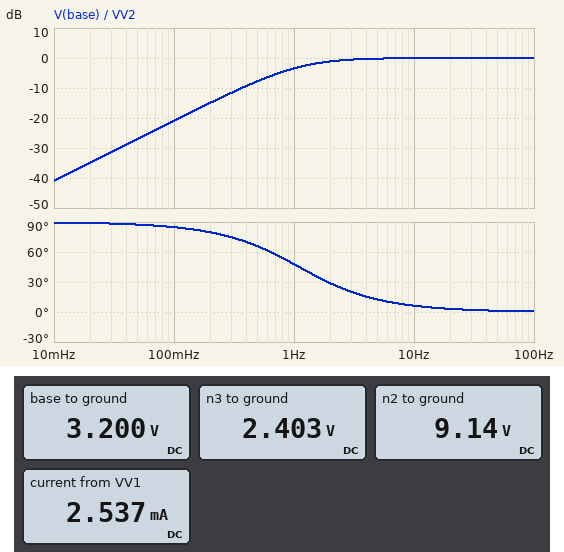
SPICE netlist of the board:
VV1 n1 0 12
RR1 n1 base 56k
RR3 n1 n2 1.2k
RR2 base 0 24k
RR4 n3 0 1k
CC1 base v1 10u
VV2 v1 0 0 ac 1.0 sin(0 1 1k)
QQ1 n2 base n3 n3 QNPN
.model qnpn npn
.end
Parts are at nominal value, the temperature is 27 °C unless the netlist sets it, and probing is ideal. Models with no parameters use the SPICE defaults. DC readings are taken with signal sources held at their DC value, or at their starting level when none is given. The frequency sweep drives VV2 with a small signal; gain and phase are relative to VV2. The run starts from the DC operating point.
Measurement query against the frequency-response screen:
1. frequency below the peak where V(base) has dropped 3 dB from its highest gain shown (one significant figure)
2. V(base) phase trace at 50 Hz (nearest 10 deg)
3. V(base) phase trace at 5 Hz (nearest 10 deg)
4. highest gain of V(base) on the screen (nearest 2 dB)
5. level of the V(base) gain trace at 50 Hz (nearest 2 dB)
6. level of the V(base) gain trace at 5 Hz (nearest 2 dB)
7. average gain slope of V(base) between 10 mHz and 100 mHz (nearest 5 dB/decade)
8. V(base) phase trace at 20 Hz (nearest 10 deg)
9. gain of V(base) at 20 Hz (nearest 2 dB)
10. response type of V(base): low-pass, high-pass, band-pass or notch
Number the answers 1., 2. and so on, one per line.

1. 1 Hz
2. 0 deg
3. 10 deg
4. 0 dB
5. 0 dB
6. 0 dB
7. 20 dB/decade
8. 0 deg
9. 0 dB
10. high-pass
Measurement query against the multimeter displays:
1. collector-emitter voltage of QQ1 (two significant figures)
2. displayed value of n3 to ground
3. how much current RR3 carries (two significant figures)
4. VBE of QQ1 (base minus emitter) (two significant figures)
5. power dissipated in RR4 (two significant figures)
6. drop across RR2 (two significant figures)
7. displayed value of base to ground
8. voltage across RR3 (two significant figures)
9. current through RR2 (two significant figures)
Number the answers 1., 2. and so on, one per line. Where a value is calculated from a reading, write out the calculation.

1. 9.14 V - 2.403 V = 6.7 V
2. 2.403 V
3. (12 V - 9.14 V) / 1.2 kΩ = 2.4 mA
4. 3.2 V - 2.403 V = 800 mV
5. (2.403 V)^2 / 1 kΩ = 5.8 mW
6. 3.2 V = 3.2 V
7. 3.200 V
8. 12 V - 9.14 V = 2.9 V
9. (3.2 V) / 24 kΩ = 130 µA
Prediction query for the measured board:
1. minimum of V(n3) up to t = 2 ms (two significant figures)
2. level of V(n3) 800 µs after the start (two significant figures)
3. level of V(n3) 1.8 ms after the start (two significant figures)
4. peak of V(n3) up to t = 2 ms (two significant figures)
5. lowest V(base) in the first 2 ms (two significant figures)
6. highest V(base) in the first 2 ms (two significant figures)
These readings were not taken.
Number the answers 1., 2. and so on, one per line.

1. 1.4 V
2. 1.5 V
3. 1.5 V
4. 3.4 V
5. 2.2 V
6. 4.2 V
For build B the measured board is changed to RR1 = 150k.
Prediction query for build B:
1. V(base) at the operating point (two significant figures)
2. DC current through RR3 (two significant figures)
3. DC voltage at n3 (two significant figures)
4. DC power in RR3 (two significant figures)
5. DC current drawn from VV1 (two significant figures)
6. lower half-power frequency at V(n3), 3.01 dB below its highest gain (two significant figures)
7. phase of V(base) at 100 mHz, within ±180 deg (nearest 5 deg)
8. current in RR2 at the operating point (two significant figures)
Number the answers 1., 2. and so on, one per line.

1. 1.5 V
2. 730 µA
3. 740 mV
4. 640 µW
5. 800 µA
6. 920 mHz
7. 85 deg
8. 63 µA
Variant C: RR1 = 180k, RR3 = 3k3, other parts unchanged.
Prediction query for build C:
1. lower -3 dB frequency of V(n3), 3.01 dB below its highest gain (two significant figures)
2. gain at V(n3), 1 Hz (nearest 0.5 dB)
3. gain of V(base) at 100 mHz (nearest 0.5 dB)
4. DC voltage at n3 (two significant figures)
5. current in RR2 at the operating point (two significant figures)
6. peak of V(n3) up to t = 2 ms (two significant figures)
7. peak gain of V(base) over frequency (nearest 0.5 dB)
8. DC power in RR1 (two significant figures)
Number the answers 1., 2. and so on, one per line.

1. 900 mHz
2. -3.0 dB
3. -19.0 dB
4. 540 mV
5. 54 µA
6. 1.5 V
7. 0 dB
8. 640 µW
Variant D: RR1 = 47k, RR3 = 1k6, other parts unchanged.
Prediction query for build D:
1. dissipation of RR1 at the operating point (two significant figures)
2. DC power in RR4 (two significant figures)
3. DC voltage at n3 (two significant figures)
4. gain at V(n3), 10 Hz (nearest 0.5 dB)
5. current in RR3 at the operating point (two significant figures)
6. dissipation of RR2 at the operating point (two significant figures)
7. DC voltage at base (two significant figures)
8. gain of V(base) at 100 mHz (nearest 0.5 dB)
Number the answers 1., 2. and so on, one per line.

1. 1.5 mW
2. 7.9 mW
3. 2.8 V
4. 0 dB
5. 2.8 mA
6. 540 µW
7. 3.6 V
8. -21.5 dB
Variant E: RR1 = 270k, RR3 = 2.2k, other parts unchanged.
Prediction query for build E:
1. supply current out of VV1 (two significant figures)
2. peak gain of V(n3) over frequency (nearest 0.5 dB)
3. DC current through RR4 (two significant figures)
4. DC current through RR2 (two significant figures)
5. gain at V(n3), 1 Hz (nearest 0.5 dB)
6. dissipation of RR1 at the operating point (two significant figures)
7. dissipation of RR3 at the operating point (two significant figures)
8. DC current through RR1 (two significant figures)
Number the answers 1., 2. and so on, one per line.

1. 240 µA
2. -1.0 dB
3. 200 µA
4. 39 µA
5. -3.5 dB
6. 450 µW
7. 89 µW
8. 41 µA
